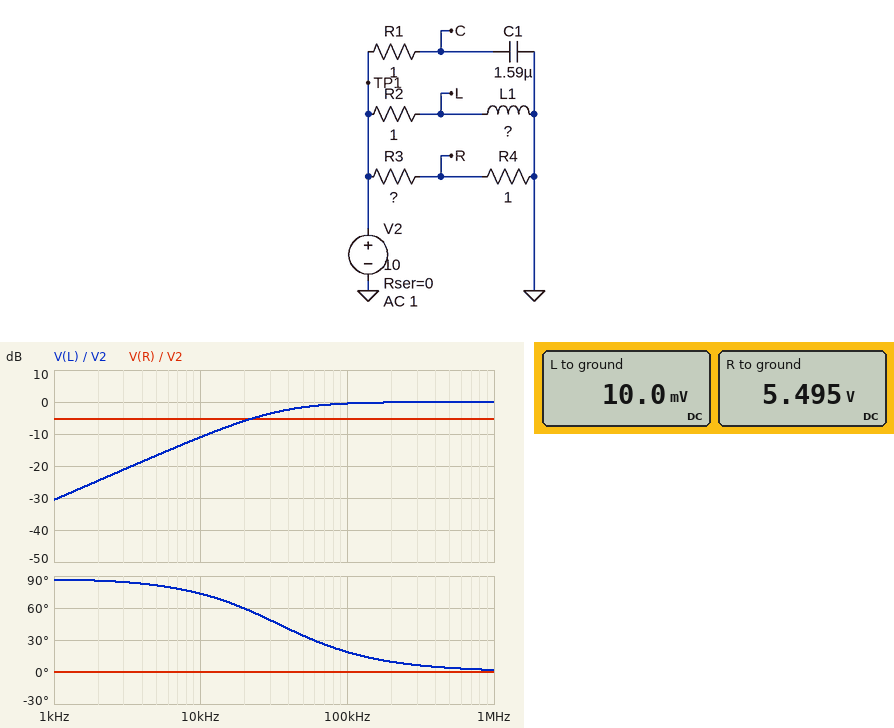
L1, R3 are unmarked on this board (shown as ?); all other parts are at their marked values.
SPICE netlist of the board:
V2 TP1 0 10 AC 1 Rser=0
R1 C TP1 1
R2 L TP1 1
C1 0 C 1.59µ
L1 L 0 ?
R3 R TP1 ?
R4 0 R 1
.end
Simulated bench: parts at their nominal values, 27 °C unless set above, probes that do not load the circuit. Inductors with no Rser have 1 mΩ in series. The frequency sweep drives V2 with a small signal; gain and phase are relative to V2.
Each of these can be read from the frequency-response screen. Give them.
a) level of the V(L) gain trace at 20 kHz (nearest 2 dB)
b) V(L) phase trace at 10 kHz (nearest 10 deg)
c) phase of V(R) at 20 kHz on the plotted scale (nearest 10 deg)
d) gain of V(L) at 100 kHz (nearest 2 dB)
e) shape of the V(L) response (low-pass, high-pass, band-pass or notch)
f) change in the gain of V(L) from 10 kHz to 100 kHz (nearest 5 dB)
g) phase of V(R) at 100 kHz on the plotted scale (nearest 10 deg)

-6 dB
70 deg
0 deg
0 dB
high-pass
10 dB
0 deg
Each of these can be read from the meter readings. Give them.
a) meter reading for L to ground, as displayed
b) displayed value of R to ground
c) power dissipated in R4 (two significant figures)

10.0 mV
5.495 V
30 W
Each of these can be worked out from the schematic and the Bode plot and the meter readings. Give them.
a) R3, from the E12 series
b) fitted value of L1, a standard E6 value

0.82 Ω
4.7 µH
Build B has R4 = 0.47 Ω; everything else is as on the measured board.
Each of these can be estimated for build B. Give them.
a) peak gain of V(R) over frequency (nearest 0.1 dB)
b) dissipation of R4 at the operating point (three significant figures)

-8.8 dB
28.2 W
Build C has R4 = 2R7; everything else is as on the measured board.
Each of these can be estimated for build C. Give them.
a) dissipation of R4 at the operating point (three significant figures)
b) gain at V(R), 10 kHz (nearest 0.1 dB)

21.8 W
-2.3 dB
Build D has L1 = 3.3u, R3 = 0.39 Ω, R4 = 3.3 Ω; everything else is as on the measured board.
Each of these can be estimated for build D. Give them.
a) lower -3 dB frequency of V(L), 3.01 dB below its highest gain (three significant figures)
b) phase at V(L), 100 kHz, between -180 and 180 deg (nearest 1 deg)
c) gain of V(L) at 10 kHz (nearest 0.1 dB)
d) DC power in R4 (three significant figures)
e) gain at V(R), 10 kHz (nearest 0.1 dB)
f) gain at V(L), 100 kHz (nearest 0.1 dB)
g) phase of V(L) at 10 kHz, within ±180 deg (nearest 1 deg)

48.3 kHz
26 deg
-13.9 dB
24.2 W
-1.0 dB
-0.9 dB
78 deg
